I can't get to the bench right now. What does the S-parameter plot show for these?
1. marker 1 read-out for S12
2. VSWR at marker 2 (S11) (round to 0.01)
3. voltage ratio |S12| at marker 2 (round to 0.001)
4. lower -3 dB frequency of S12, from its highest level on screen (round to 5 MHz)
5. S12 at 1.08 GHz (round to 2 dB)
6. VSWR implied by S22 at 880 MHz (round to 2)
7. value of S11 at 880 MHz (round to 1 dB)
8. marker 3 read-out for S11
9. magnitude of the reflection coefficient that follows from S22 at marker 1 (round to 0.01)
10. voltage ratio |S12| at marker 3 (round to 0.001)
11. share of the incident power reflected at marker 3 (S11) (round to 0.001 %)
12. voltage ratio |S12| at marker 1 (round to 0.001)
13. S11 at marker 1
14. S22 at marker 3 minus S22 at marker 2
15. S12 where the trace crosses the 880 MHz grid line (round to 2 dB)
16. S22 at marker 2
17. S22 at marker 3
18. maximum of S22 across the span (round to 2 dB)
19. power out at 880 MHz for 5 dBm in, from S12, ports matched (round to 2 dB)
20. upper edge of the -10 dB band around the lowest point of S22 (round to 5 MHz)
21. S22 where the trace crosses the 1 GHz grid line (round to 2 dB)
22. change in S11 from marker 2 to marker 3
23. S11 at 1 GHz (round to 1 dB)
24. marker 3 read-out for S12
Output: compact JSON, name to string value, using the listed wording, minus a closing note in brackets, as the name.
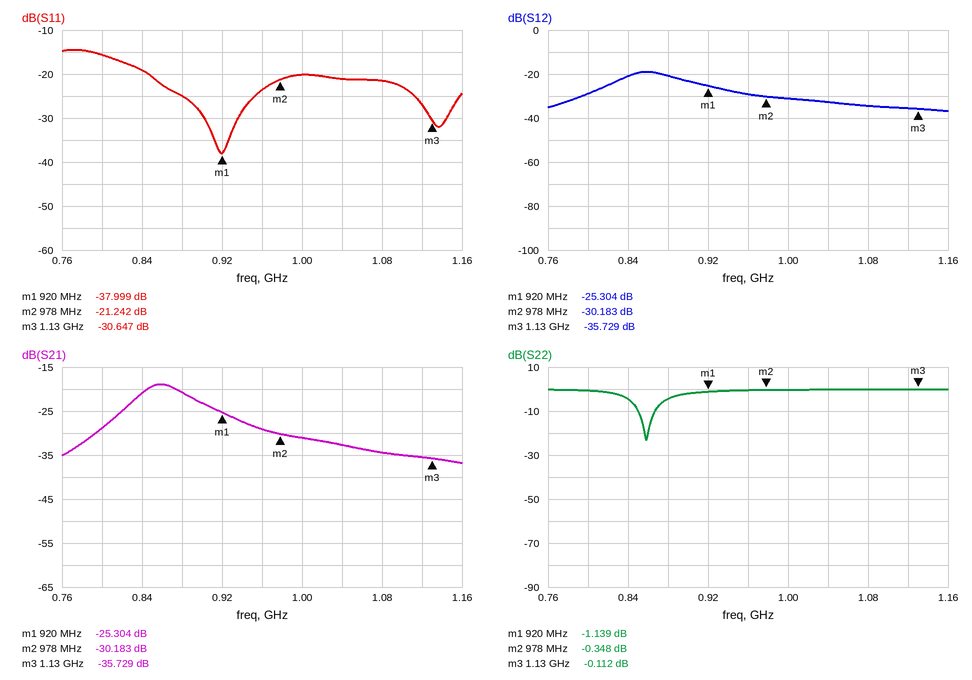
{"marker 1 read-out for S12": "-25.304 dB", "VSWR at marker 2 (S11)": "1.19", "voltage ratio |S12| at marker 2": "0.031", "lower -3 dB frequency of S12, from its highest level on screen": "835 MHz", "S12 at 1.08 GHz": "-34 dB", "VSWR implied by S22 at 880 MHz": "4", "value of S11 at 880 MHz": "-25 dB", "marker 3 read-out for S11": "-30.647 dB", "magnitude of the reflection coefficient that follows from S22 at marker 1": "0.88", "voltage ratio |S12| at marker 3": "0.016", "share of the incident power reflected at marker 3 (S11)": "0.086 %", "voltage ratio |S12| at marker 1": "0.054", "S11 at marker 1": "-37.999 dB", "S22 at marker 3 minus S22 at marker 2": "0.236 dB", "S12 where the trace crosses the 880 MHz grid line": "-20 dB", "S22 at marker 2": "-0.348 dB", "S22 at marker 3": "-0.112 dB", "maximum of S22 across the span": "0 dB", "power out at 880 MHz for 5 dBm in, from S12, ports matched": "-16 dBm", "upper edge of the -10 dB band around the lowest point of S22": "865 MHz", "S22 where the trace crosses the 1 GHz grid line": "0 dB", "change in S11 from marker 2 to marker 3": "-9.405 dB", "S11 at 1 GHz": "-20 dB", "marker 3 read-out for S12": "-35.729 dB"}
